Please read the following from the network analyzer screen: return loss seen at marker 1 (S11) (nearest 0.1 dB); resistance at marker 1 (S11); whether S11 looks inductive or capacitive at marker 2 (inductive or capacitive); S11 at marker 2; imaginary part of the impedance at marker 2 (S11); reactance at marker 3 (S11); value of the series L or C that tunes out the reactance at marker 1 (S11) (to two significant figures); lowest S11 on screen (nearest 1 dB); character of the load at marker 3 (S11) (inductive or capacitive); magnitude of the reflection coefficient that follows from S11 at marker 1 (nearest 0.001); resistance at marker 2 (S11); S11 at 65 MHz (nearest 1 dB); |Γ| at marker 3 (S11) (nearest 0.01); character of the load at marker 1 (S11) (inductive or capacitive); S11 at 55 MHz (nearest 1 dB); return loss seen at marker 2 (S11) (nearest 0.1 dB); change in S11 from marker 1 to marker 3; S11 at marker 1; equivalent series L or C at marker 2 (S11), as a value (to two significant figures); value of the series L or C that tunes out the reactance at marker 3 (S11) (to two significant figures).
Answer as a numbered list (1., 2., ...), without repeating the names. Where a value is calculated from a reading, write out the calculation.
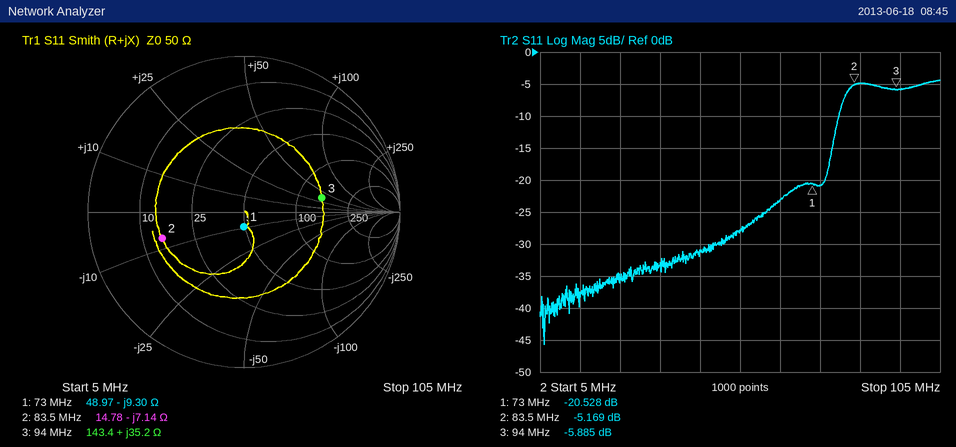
1. 20.5 dB
2. 48.97 Ω
3. capacitive
4. -5.169 dB
5. -7.14 Ω
6. +35.2 Ω
7. L = 9.3 Ω/(2π × 73 MHz) ≈ 20 nH
8. -46 dB
9. inductive
10. 10^(-20.528/20) ≈ 0.094
11. 14.78 Ω
12. -23 dB
13. 0.51
14. capacitive
15. -28 dB
16. 5.2 dB
17. -5.885 − (-20.528) = 14.643 dB
18. -20.528 dB
19. C = 1/(2π × 83.5 MHz × 7.14 Ω) ≈ 267 pF, so 270 pF to two significant figures
20. C = 1/(2π × 94 MHz × 35.2 Ω) ≈ 48 pF
